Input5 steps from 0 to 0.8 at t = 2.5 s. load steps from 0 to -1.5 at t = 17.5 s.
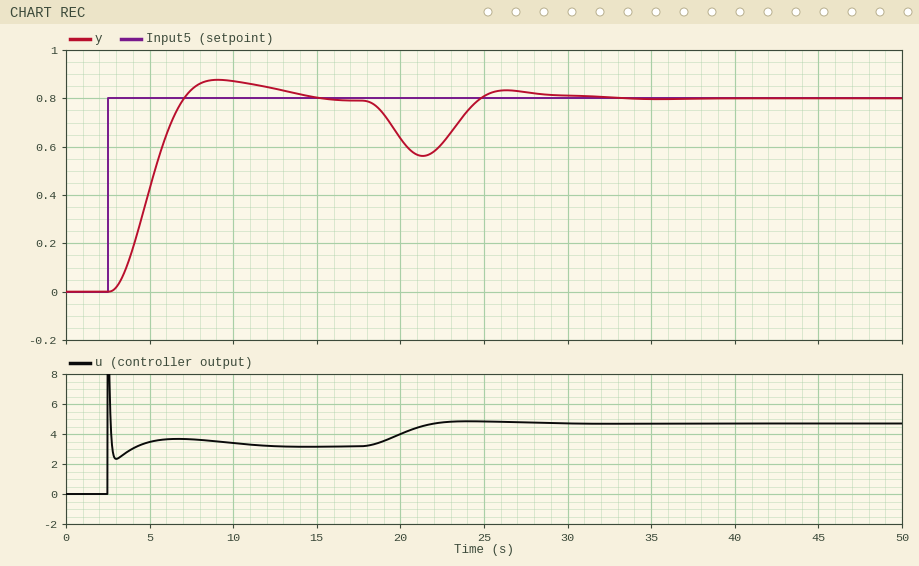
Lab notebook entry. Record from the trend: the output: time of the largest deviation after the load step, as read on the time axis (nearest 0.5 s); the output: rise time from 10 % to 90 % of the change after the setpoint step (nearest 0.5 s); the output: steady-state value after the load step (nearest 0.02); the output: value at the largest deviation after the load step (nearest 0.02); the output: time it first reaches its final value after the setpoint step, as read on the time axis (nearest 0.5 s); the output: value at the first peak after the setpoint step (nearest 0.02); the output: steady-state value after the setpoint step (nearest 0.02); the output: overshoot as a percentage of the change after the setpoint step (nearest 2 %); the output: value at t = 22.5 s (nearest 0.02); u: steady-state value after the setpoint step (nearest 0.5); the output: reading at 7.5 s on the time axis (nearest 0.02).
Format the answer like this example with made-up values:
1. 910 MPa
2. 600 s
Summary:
1. 21.5 s
2. 3.0 s
3. 0.80
4. 0.56
5. 7.0 s
6. 0.88
7. 0.80
8. 10 %
9. 0.62
10. 3.0
11. 0.84
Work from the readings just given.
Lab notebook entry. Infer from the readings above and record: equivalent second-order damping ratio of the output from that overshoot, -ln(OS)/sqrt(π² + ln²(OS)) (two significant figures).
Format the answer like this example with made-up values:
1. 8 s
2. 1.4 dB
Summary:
1. 0.59
